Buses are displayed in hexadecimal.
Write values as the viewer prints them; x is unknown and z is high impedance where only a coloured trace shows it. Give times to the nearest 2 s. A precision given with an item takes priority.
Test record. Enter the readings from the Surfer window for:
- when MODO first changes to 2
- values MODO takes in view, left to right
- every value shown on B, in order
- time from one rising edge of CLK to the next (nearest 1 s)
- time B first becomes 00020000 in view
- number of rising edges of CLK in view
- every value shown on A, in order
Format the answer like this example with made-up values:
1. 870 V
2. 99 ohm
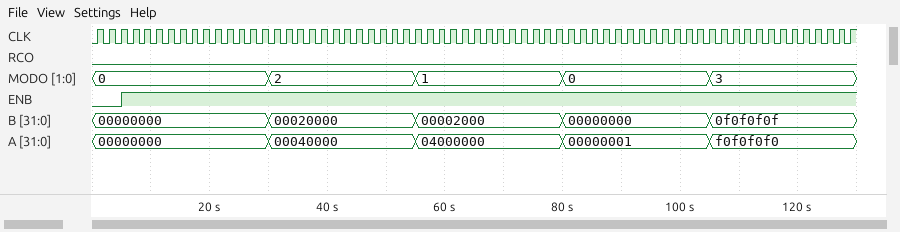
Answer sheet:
1. 30 s
2. 0, 2, 1, 0, 3
3. 00000000, 00020000, 00002000, 00000000, 0f0f0f0f
4. 2 s
5. 30 s
6. 65
7. 00000000, 00040000, 04000000, 00000001, f0f0f0f0
